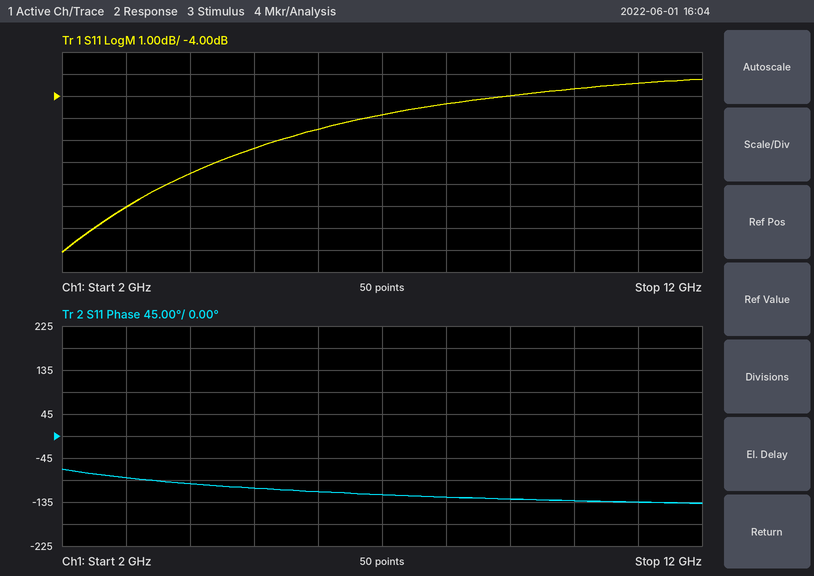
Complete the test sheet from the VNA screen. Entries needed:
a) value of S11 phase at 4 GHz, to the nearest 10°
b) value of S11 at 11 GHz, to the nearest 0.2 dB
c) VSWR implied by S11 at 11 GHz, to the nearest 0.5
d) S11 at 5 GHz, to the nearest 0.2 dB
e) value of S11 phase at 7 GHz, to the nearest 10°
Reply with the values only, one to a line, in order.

-100°
-3.4 dB
5.0
-6.4 dB
-120°
